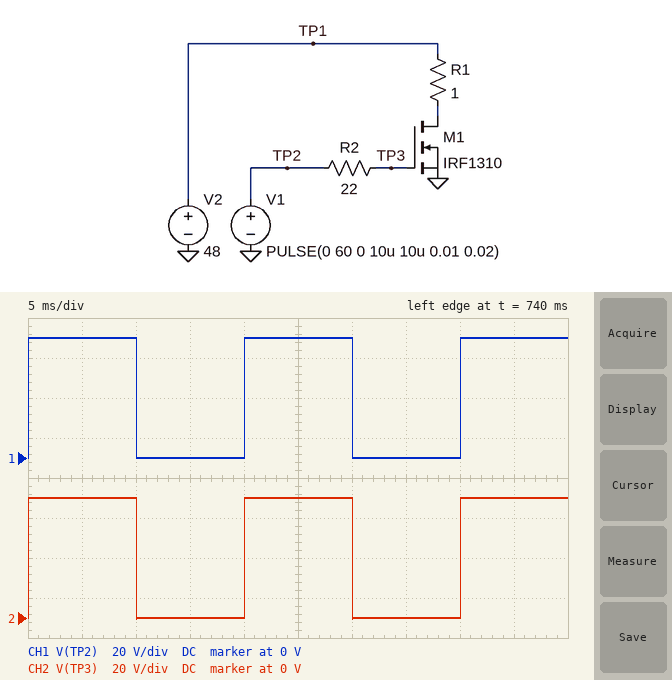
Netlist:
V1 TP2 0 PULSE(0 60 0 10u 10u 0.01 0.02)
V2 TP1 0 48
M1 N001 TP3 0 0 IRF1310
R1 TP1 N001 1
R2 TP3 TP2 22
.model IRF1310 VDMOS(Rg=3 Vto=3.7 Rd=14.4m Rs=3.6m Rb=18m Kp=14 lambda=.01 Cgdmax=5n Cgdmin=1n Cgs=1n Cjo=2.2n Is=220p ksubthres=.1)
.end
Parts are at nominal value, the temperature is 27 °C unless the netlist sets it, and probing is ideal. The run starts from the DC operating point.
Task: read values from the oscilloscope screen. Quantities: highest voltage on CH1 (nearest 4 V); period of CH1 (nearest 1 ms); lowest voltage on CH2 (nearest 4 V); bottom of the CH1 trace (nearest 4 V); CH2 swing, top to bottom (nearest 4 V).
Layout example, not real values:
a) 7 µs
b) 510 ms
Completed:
a) 60 V
b) 20 ms
c) 0 V
d) 0 V
e) 60 V
